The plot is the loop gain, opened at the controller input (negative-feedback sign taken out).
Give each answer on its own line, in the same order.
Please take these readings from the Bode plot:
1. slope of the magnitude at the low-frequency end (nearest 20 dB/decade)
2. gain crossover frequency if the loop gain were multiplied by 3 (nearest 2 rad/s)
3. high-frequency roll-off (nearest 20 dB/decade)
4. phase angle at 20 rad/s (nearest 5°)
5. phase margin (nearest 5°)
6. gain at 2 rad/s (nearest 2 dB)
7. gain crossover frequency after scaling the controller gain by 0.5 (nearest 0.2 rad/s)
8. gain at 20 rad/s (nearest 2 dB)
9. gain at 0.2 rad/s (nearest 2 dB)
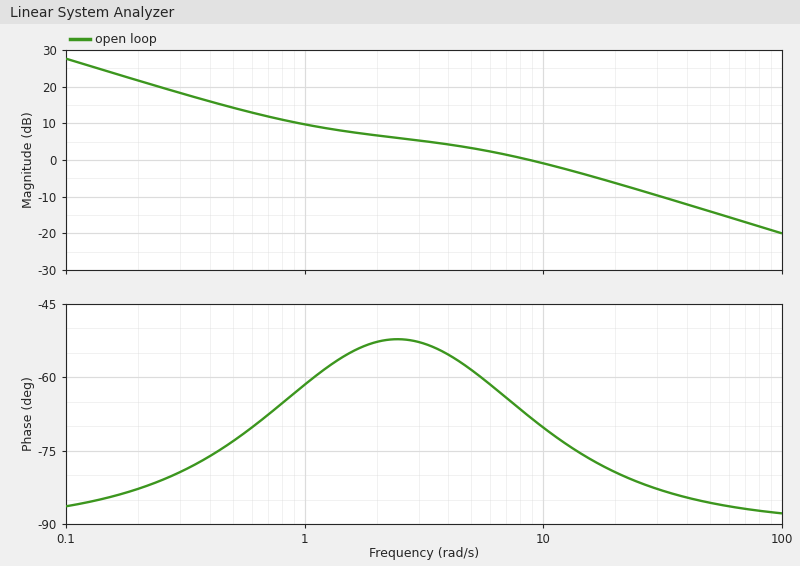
-20 dB/decade
30 rad/s
-20 dB/decade
-80°
110°
6 dB
2.4 rad/s
-6 dB
22 dB
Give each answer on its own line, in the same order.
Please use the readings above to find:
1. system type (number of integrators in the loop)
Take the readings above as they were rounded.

1
